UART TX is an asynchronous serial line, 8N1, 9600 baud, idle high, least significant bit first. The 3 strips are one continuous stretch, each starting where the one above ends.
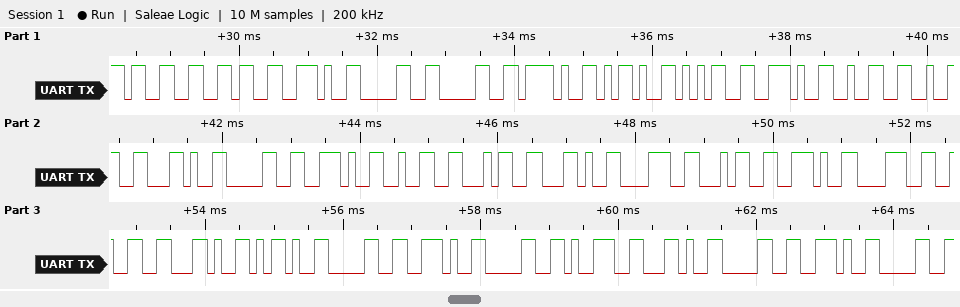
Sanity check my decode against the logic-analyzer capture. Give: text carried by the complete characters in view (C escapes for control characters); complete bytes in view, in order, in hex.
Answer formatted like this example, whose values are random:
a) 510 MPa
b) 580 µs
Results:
a) "36.00/-5.22,0.24,84.82,-0.09,0.0"
b) 33 36 2E 30 30 2F 2D 35 2E 32 32 2C 30 2E 32 34 2C 38 34 2E 38 32 2C 2D 30 2E 30 39 2C 30 2E 30
